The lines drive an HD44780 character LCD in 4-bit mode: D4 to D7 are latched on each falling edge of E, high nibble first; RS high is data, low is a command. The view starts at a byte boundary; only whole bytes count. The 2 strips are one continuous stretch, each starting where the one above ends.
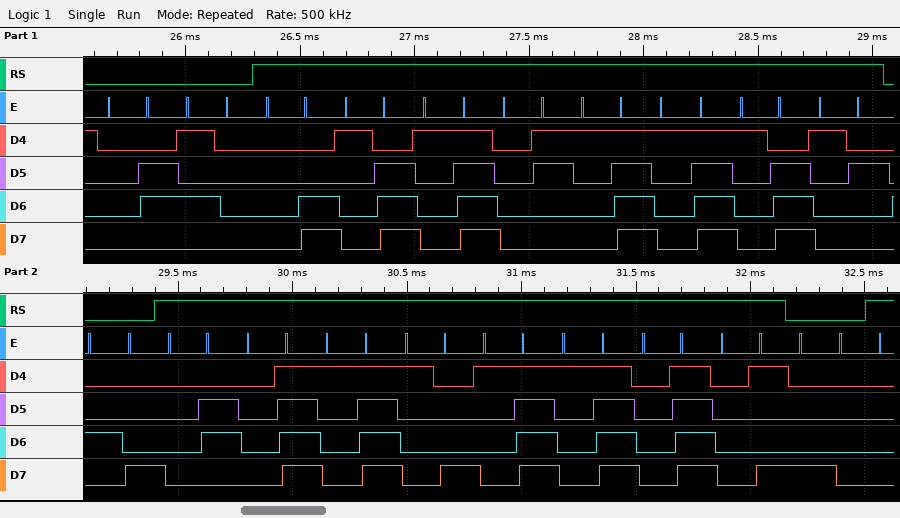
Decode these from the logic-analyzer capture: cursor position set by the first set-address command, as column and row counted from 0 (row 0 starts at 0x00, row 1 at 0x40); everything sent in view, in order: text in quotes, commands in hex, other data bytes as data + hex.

column 0, row 0
0x06 0x50 data 0C 1E 1F 03 1F 1F 1E 12 0x48 data 06 0F 1F 18 1F 1F 0F 09 0x80
